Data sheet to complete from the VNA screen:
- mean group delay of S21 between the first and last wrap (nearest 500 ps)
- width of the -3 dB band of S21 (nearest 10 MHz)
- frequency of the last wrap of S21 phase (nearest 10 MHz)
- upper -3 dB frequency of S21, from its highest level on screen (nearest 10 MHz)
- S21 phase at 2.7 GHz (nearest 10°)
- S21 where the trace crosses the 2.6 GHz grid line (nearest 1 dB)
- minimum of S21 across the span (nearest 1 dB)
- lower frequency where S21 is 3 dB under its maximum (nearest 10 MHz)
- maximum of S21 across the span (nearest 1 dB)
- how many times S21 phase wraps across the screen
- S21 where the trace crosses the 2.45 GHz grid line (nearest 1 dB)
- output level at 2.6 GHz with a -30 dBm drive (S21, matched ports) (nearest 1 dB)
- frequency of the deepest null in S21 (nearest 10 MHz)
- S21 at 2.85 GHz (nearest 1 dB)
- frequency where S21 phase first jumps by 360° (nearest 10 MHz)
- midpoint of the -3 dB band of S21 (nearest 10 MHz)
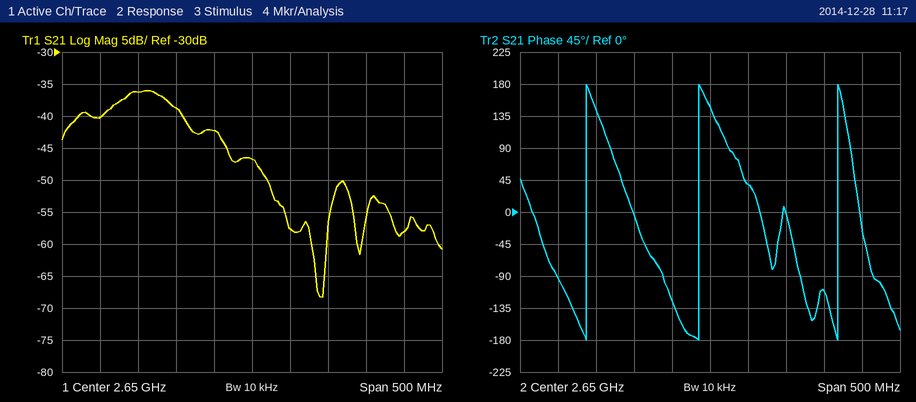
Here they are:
6.0 ns
90 MHz
2.82 GHz
2.55 GHz
40°
-42 dB
-68 dB
2.46 GHz
-36 dB
3
-40 dB
-72 dBm
2.74 GHz
-58 dB
2.49 GHz
2.51 GHz
